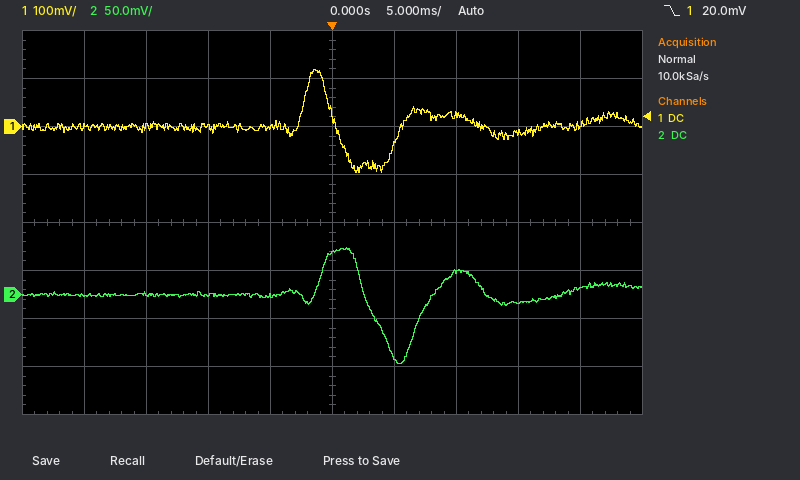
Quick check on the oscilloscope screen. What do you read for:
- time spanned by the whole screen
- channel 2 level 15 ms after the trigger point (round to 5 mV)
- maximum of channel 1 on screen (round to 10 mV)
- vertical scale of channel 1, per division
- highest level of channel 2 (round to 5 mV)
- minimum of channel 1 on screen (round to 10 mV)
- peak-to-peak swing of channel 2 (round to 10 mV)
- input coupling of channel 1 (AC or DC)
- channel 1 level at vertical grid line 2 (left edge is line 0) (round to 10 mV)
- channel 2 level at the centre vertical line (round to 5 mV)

50 ms
-10 mV
120 mV
100 mV
50 mV
-100 mV
120 mV
DC
0 mV
45 mV
